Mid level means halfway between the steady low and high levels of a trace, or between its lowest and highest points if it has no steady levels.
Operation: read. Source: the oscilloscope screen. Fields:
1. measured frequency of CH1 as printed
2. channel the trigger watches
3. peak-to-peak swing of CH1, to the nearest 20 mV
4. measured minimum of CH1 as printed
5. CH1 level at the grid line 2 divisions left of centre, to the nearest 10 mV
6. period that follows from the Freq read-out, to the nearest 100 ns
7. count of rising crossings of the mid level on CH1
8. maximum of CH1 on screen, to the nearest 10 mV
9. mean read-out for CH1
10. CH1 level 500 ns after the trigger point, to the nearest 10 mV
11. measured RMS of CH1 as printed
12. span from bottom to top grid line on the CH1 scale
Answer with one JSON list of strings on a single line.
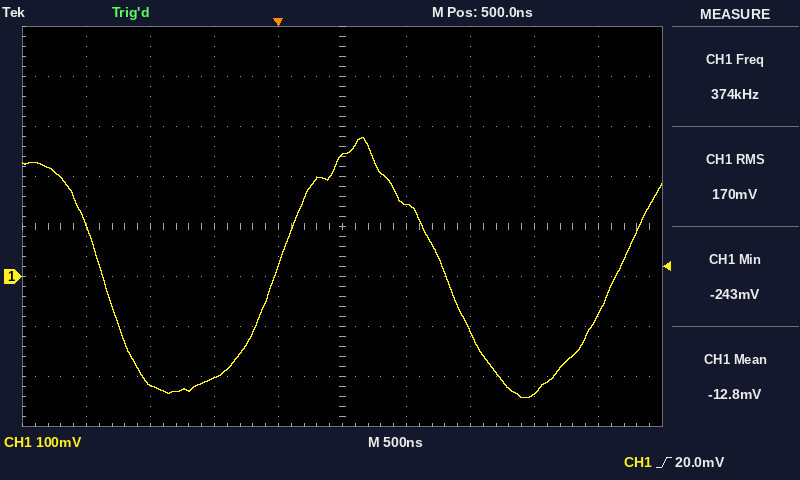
["374 kHz", "CH1", "520 mV", "-243 mV", "-200 mV", "2.7 µs", "2", "280 mV", "-12.8 mV", "240 mV", "170 mV", "800 mV"]
